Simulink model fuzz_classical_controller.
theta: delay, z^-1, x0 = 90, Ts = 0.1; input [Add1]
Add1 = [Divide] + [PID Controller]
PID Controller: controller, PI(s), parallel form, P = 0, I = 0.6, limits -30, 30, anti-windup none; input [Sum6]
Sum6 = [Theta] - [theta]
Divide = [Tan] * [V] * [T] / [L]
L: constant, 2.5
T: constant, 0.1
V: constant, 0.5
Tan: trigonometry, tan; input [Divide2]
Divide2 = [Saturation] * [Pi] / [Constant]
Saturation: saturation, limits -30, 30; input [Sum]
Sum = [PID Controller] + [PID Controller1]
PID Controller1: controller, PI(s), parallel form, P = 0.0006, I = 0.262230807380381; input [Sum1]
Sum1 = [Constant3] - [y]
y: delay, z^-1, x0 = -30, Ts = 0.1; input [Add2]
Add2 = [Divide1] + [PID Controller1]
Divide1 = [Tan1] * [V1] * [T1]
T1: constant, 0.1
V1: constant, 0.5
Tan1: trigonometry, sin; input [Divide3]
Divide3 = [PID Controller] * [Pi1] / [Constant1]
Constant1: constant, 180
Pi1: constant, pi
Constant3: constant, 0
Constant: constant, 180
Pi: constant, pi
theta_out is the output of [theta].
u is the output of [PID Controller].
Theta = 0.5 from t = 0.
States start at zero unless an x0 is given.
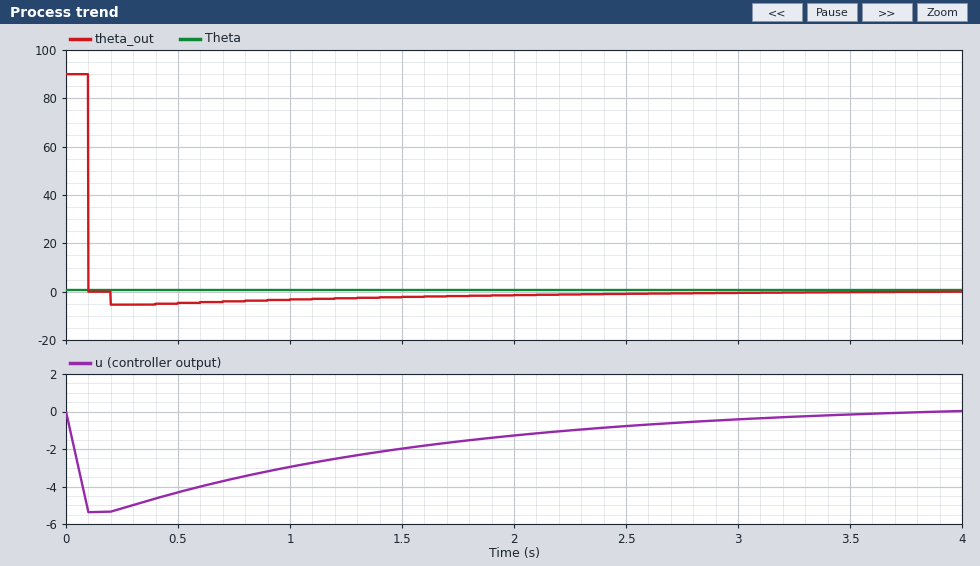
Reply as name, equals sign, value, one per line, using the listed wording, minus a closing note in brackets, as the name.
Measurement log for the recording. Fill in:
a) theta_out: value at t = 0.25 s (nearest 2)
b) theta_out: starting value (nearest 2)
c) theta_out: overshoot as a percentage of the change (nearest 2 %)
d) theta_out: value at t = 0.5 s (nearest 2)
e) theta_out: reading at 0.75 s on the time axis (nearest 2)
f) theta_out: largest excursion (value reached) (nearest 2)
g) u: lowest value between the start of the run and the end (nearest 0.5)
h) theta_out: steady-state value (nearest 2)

theta_out: value at t = 0.25 s = -6
theta_out: starting value = 90
theta_out: overshoot as a percentage of the change = 6 %
theta_out: value at t = 0.5 s = -4
theta_out: reading at 0.75 s on the time axis = -4
theta_out: largest excursion (value reached) = -6
u: lowest value between the start of the run and the end = -5.5
theta_out: steady-state value = 0
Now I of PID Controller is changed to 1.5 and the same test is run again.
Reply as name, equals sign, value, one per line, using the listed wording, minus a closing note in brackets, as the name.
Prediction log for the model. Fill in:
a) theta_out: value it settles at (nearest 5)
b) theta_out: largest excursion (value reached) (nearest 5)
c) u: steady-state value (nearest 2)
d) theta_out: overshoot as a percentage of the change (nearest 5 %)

theta_out: value it settles at = 0
theta_out: largest excursion (value reached) = -15
u: steady-state value = 0
theta_out: overshoot as a percentage of the change = 15 %
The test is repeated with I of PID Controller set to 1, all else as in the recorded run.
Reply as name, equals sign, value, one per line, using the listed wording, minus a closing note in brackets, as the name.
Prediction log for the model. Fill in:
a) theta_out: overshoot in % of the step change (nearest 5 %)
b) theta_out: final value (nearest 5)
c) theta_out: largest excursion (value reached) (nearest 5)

theta_out: overshoot in % of the step change = 10 %
theta_out: final value = 0
theta_out: largest excursion (value reached) = -10
